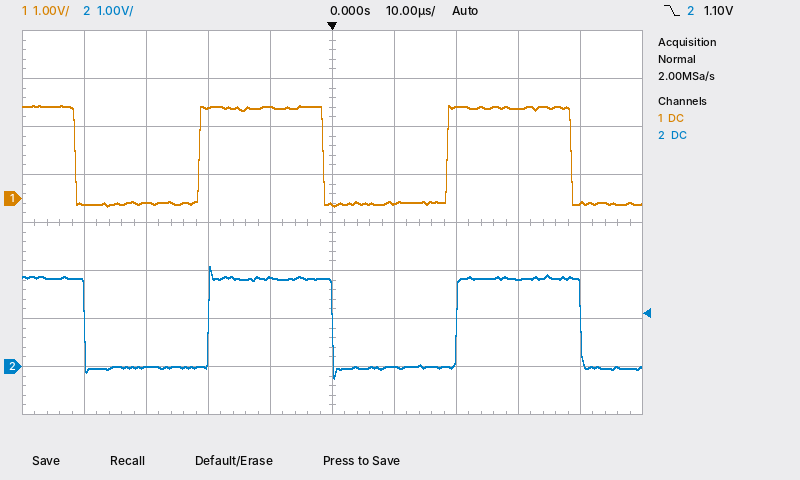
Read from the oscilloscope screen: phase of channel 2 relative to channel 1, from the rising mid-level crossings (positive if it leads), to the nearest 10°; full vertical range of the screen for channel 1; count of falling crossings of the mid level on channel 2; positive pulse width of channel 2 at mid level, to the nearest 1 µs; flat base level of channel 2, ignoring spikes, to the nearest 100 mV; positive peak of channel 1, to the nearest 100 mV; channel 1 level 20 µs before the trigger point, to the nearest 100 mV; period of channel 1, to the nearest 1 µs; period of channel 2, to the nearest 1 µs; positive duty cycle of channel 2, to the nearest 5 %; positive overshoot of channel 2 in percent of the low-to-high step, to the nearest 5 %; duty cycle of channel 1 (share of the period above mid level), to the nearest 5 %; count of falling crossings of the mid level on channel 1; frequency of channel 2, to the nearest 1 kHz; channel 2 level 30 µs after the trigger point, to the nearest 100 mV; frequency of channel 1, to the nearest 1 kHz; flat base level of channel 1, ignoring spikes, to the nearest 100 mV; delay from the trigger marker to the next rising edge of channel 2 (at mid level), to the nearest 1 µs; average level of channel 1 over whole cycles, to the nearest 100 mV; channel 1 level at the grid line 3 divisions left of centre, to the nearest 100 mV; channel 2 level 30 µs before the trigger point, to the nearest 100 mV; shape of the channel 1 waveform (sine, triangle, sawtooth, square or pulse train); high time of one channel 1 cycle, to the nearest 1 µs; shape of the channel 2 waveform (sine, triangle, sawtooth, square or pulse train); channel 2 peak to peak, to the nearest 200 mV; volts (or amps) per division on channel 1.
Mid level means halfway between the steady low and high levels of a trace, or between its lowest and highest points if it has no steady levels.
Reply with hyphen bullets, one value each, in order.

- -10°
- 8 V
- 3
- 20 µs
- 0.0 V
- 1.9 V
- 1.9 V
- 40 µs
- 40 µs
- 50 %
- 15 %
- 50 %
- 3
- 25 kHz
- 1.8 V
- 25 kHz
- -100 mV
- 20 µs
- 900 mV
- -100 mV
- 0.0 V
- square
- 20 µs
- square
- 2.4 V
- 1 V
